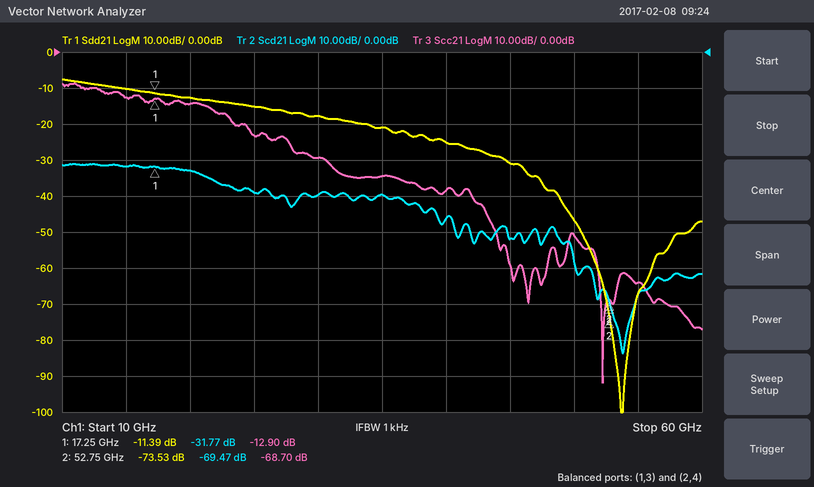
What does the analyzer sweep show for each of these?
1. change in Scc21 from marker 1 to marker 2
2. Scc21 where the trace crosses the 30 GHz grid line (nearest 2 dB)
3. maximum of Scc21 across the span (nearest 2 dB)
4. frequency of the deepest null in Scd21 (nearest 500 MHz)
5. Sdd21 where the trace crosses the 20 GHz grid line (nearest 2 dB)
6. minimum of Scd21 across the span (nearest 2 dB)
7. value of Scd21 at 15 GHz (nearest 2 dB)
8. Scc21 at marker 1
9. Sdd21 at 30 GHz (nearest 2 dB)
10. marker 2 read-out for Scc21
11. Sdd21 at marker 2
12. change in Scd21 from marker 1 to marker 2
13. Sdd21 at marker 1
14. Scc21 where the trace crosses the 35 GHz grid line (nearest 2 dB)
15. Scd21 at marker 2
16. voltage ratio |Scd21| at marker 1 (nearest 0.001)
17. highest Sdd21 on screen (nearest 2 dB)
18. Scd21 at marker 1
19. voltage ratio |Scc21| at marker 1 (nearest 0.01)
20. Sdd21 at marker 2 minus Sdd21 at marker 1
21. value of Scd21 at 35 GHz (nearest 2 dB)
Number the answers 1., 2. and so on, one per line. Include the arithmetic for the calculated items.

1. -68.7 − (-12.9) = -55.80 dB
2. -30 dB
3. -8 dB
4. 54.0 GHz
5. -12 dB
6. -84 dB
7. -32 dB
8. -12.90 dB
9. -18 dB
10. -68.70 dB
11. -73.53 dB
12. -69.47 − (-31.77) = -37.70 dB
13. -11.39 dB
14. -34 dB
15. -69.47 dB
16. 10^(-31.77/20) ≈ 0.026
17. -8 dB
18. -31.77 dB
19. 10^(-12.9/20) ≈ 0.23
20. -73.53 − (-11.39) = -62.14 dB
21. -40 dB
